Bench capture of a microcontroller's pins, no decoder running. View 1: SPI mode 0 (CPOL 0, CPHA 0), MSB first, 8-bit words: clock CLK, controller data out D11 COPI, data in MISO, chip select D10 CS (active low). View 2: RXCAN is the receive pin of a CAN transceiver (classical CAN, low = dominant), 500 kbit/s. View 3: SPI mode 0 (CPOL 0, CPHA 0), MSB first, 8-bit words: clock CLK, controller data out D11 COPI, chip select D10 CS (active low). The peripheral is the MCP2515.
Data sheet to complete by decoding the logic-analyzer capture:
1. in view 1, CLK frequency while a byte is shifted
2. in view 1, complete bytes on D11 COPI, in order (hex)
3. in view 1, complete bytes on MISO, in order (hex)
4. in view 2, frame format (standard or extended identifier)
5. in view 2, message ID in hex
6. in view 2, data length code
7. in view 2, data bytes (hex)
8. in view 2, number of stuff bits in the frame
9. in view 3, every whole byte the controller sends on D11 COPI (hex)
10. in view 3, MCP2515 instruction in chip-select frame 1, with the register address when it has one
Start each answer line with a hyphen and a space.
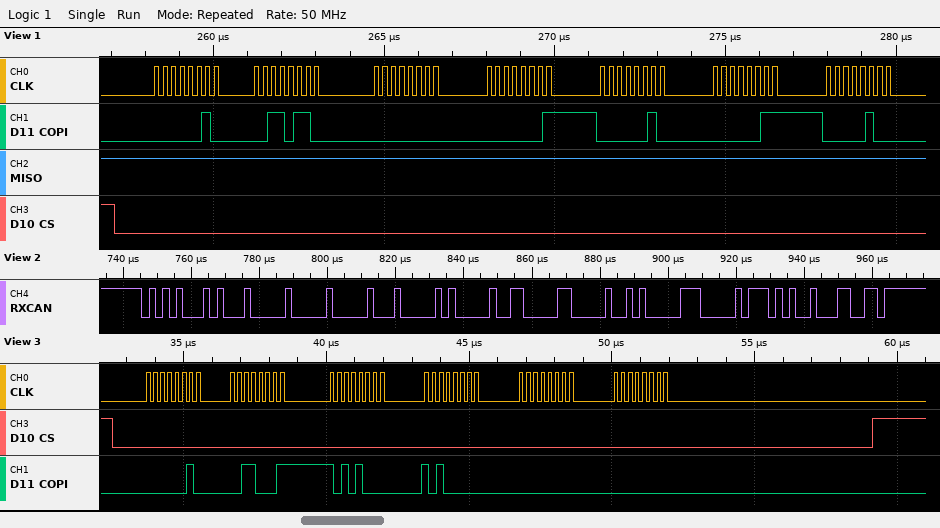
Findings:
- 4 MHz
- 02 36 00 01 02 03 04
- FF FF FF FF FF FF FF
- standard
- 0x545
- 8
- 00 01 02 03 04 05 06 07
- 9
- 0x02 0x31 0xA8 0xA0 0x00 0x00
- WRITE 0x31
